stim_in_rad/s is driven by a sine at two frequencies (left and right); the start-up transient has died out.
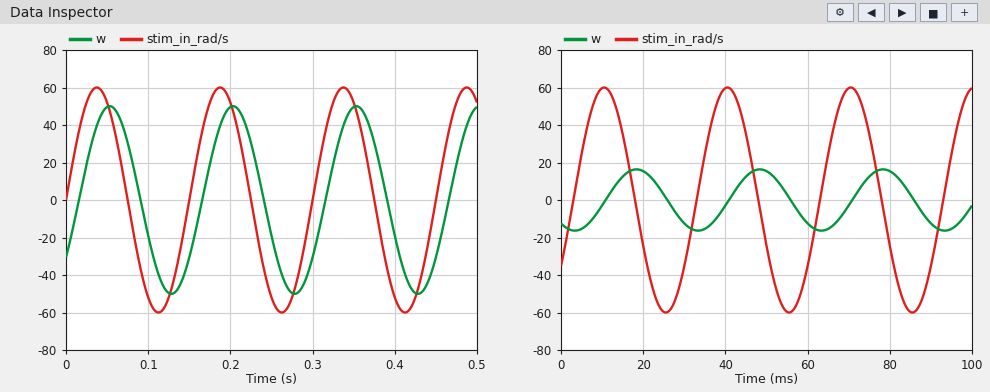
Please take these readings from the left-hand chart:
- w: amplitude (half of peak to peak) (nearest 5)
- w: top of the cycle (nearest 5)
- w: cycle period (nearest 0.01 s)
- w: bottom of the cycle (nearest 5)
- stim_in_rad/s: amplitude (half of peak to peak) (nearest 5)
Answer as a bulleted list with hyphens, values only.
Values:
- 50
- 50
- 0.15 s
- -50
- 60
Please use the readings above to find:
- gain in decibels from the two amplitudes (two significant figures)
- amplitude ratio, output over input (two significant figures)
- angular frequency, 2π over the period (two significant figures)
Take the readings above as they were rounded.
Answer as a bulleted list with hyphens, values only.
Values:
- -1.6 dB
- 0.83
- 42 rad/s
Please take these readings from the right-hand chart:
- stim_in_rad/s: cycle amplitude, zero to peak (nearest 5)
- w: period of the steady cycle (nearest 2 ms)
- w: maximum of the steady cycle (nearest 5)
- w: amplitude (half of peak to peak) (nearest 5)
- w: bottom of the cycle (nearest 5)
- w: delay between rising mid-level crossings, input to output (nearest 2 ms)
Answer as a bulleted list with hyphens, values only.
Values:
- 60
- 30 ms
- 15
- 15
- -15
- 8 ms
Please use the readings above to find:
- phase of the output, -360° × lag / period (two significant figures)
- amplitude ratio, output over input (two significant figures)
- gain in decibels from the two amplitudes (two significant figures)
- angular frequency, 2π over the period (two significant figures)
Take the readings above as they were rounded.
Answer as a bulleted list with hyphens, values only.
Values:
- -96°
- 0.25
- -12 dB
- 0.21 rad/ms
